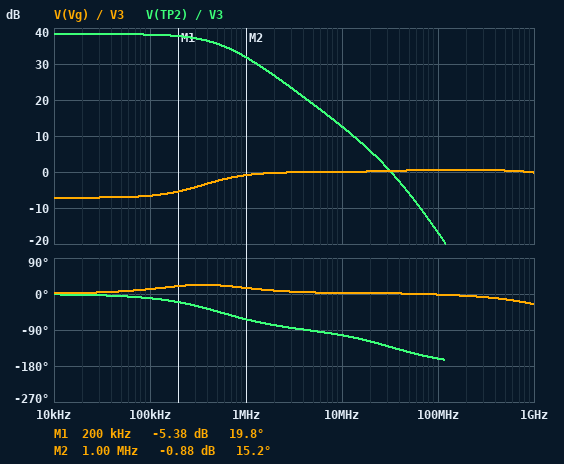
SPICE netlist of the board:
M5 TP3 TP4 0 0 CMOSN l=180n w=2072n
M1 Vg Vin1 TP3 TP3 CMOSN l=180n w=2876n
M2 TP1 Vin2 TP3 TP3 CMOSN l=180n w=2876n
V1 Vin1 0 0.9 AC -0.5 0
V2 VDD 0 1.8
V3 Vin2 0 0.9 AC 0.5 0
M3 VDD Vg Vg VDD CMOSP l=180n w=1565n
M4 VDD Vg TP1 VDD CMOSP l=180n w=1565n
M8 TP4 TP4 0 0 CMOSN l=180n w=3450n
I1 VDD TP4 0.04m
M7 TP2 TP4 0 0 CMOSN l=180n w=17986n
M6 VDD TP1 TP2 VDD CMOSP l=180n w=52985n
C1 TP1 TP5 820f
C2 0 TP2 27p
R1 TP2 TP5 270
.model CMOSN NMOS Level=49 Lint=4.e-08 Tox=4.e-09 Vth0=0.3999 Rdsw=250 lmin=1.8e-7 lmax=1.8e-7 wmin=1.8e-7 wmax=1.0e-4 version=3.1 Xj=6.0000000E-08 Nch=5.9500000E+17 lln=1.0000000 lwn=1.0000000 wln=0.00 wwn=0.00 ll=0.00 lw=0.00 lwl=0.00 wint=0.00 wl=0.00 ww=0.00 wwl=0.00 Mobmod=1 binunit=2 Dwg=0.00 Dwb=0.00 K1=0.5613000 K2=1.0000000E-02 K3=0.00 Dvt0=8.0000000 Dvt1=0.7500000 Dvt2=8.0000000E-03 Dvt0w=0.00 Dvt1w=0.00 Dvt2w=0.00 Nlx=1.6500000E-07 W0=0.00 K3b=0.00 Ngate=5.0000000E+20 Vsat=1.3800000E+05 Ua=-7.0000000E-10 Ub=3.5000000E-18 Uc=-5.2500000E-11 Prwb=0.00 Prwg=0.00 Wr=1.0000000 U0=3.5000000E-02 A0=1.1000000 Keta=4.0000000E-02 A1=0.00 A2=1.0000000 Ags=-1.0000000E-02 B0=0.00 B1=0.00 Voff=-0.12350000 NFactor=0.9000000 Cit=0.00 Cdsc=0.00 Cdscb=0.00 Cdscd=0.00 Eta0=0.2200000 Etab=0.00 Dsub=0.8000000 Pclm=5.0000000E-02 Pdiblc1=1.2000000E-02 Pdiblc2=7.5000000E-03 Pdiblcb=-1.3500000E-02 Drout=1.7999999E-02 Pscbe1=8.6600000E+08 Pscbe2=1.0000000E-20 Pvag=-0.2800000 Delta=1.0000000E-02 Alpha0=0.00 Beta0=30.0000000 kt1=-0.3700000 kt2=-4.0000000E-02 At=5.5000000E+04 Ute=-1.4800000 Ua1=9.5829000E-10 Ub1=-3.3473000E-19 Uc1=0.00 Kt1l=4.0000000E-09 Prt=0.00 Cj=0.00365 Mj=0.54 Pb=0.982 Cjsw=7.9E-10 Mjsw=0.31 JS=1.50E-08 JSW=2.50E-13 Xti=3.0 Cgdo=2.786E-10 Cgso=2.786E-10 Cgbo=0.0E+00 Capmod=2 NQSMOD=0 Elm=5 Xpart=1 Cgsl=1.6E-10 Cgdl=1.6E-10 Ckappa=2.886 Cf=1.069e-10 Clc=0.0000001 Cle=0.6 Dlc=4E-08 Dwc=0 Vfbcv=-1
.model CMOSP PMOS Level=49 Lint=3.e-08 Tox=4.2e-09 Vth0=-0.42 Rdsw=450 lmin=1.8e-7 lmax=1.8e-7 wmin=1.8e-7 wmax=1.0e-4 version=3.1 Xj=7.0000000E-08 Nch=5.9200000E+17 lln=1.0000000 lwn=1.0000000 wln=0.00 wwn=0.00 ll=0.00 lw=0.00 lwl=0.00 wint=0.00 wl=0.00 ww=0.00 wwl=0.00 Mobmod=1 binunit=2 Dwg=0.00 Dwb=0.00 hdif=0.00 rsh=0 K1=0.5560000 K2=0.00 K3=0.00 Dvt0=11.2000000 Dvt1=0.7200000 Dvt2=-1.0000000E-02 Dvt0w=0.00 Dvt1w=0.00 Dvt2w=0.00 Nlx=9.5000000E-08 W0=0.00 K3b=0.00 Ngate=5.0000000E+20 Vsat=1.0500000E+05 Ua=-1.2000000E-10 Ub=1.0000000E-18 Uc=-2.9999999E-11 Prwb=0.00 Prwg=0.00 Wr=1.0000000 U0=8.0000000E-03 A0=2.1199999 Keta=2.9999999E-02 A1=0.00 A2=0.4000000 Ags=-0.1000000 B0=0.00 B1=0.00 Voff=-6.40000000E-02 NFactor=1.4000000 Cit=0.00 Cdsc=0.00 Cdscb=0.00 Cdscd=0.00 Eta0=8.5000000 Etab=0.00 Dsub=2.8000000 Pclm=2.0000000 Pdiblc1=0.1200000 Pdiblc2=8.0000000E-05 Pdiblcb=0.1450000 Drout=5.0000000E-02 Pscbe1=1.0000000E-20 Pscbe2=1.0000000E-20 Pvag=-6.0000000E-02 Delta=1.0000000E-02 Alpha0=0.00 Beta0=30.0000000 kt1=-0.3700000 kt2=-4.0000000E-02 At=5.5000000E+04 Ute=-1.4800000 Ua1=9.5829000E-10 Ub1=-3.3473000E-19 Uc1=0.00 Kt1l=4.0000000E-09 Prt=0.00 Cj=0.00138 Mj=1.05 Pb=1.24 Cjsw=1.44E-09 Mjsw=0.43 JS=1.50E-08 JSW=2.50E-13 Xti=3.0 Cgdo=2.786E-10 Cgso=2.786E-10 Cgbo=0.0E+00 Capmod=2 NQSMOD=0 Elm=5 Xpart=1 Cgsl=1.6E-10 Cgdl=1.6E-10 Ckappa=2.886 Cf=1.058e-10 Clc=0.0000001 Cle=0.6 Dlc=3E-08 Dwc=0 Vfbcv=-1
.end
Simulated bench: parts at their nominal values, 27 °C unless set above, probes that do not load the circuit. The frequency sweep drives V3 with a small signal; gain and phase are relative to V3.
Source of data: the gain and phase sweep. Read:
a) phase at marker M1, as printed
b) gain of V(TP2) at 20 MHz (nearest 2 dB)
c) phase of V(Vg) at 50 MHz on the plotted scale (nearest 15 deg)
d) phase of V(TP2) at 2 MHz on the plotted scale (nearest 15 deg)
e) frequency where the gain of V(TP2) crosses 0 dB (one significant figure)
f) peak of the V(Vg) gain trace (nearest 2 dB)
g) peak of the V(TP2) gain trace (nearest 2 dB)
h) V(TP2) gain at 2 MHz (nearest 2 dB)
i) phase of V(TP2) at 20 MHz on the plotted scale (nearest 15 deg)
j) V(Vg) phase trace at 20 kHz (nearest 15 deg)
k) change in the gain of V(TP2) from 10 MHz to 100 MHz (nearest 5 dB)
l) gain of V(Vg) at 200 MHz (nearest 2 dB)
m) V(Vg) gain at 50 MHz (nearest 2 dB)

19.8 deg
6 dB
0 deg
-75 deg
30 MHz
0 dB
38 dB
26 dB
-120 deg
0 deg
-30 dB
0 dB
0 dB
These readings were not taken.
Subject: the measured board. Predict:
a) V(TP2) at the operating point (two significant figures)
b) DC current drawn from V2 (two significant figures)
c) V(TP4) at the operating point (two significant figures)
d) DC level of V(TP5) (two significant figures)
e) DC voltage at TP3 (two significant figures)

1.3 V
520 µA
480 mV
1.3 V
510 mV
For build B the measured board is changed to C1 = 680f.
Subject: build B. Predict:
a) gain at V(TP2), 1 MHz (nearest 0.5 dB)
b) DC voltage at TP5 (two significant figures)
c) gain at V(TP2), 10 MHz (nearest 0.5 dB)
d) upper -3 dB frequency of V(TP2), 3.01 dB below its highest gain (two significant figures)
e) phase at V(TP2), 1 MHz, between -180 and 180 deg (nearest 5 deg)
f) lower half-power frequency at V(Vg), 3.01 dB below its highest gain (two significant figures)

33.0 dB
1.3 V
14.0 dB
630 kHz
-60 deg
610 kHz
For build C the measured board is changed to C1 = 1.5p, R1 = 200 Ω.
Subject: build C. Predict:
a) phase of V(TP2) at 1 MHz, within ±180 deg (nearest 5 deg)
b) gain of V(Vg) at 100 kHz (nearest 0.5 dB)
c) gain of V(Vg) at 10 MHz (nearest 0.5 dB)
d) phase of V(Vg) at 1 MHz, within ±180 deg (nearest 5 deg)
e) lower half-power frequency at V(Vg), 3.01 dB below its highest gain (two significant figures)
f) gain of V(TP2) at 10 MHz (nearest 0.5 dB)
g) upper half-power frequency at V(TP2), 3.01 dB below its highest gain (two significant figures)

-75 deg
-5.5 dB
0.5 dB
10 deg
280 kHz
8.0 dB
320 kHz
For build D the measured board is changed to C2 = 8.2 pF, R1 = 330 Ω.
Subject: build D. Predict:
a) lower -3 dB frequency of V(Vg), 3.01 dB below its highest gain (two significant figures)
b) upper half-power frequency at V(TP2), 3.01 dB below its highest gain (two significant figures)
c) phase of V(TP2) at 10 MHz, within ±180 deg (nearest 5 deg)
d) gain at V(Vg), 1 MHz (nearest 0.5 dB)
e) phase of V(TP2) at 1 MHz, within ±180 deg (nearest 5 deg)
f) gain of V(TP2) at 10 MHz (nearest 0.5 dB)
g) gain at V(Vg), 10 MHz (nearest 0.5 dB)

490 kHz
590 kHz
-90 deg
-0.5 dB
-60 deg
13.5 dB
0.5 dB
